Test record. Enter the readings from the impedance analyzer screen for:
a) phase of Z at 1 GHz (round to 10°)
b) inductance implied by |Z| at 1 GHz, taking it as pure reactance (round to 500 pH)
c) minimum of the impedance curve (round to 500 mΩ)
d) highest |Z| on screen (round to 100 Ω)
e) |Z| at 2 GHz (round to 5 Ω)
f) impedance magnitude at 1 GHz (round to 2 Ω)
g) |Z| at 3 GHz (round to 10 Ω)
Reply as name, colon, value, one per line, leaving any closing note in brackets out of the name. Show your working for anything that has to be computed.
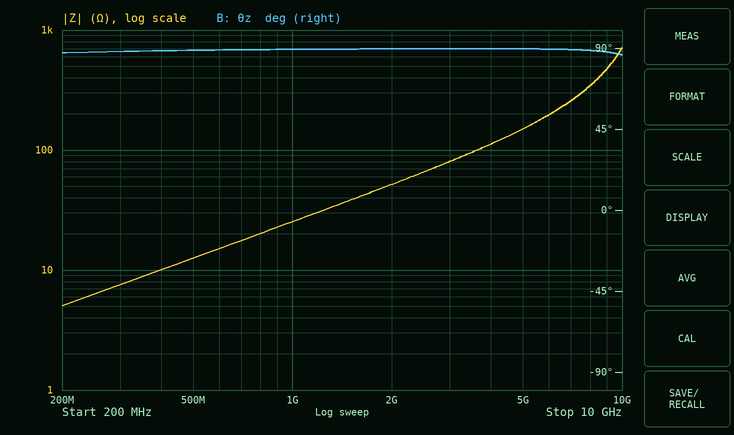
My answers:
phase of Z at 1 GHz: 90°
inductance implied by |Z| at 1 GHz, taking it as pure reactance: L = 26 Ω/(2π × 1 GHz) ≈ 4.14 nH, so 4.0 nH to the nearest 500 pH
minimum of the impedance curve: 5.0 Ω
highest |Z| on screen: 700 Ω
|Z| at 2 GHz: 50 Ω
impedance magnitude at 1 GHz: 26 Ω
|Z| at 3 GHz: 80 Ω
